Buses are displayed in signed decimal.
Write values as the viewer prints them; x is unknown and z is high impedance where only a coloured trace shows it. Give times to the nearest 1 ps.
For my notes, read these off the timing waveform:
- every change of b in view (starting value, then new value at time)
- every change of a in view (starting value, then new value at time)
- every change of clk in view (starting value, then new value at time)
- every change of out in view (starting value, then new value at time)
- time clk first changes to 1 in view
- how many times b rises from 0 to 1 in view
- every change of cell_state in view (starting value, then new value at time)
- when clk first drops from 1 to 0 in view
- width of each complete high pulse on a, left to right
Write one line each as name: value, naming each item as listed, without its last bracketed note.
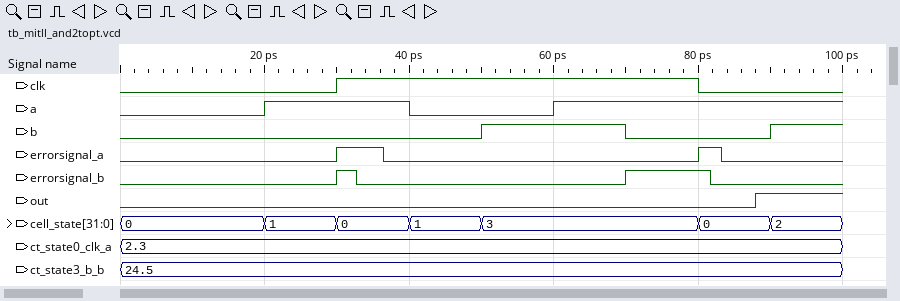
every change of b in view: 0, 1 at 50 ps, 0 at 70 ps, 1 at 90 ps
every change of a in view: 0, 1 at 20 ps, 0 at 40 ps, 1 at 60 ps
every change of clk in view: 0, 1 at 30 ps, 0 at 80 ps
every change of out in view: 0, 1 at 88 ps
time clk first changes to 1 in view: 30 ps
how many times b rises from 0 to 1 in view: 2
every change of cell_state in view: 0, 1 at 20 ps, 0 at 30 ps, 1 at 40 ps, 3 at 50 ps, 0 at 80 ps, 2 at 90 ps
when clk first drops from 1 to 0 in view: 80 ps
width of each complete high pulse on a, left to right: 20 ps
